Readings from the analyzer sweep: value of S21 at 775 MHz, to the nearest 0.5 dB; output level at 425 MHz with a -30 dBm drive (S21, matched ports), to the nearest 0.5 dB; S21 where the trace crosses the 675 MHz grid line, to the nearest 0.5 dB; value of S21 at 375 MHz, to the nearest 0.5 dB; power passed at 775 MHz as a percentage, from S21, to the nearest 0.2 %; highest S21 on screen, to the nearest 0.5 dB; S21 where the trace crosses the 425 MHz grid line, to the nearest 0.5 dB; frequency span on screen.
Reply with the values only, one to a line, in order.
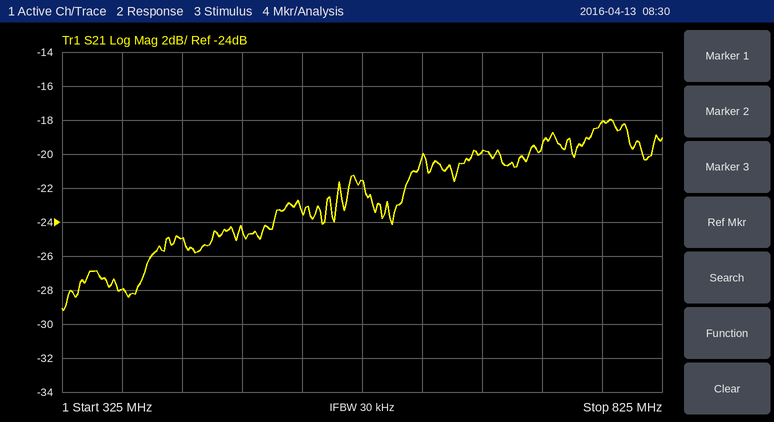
-18.0 dB
-55.0 dBm
-20.0 dB
-28.0 dB
1.6 %
-18.0 dB
-25.0 dB
500 MHz
